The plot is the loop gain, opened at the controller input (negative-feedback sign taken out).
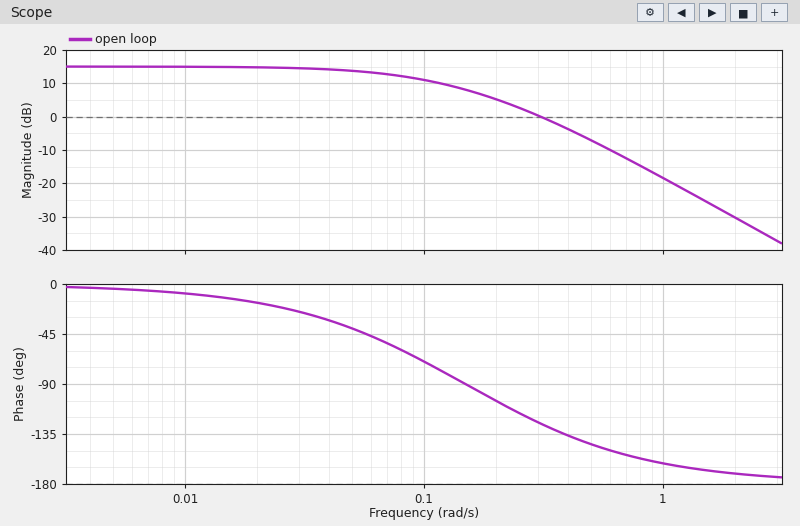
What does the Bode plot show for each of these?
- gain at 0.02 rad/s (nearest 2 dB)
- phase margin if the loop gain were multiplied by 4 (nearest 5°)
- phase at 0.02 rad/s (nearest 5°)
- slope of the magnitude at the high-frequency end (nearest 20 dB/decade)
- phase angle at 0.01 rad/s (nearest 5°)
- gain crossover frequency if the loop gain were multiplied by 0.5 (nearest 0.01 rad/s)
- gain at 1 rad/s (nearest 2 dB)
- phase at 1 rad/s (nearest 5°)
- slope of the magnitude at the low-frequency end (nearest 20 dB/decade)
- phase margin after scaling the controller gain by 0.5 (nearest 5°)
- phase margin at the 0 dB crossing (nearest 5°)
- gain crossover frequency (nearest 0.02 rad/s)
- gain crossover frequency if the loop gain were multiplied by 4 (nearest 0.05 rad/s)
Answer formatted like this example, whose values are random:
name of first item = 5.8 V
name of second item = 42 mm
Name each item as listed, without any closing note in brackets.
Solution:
gain at 0.02 rad/s = 14 dB
phase margin if the loop gain were multiplied by 4 = 25°
phase at 0.02 rad/s = -15°
slope of the magnitude at the high-frequency end = -40 dB/decade
phase angle at 0.01 rad/s = -10°
gain crossover frequency if the loop gain were multiplied by 0.5 = 0.19 rad/s
gain at 1 rad/s = -18 dB
phase at 1 rad/s = -160°
slope of the magnitude at the low-frequency end = 0 dB/decade
phase margin after scaling the controller gain by 0.5 = 80°
phase margin at the 0 dB crossing = 55°
gain crossover frequency = 0.30 rad/s
gain crossover frequency if the loop gain were multiplied by 4 = 0.70 rad/s
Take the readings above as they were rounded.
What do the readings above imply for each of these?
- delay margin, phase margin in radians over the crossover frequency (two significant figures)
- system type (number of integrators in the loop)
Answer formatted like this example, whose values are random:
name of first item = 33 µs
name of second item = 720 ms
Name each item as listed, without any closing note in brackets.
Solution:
delay margin, phase margin in radians over the crossover frequency = 3.2 s
system type = 0
